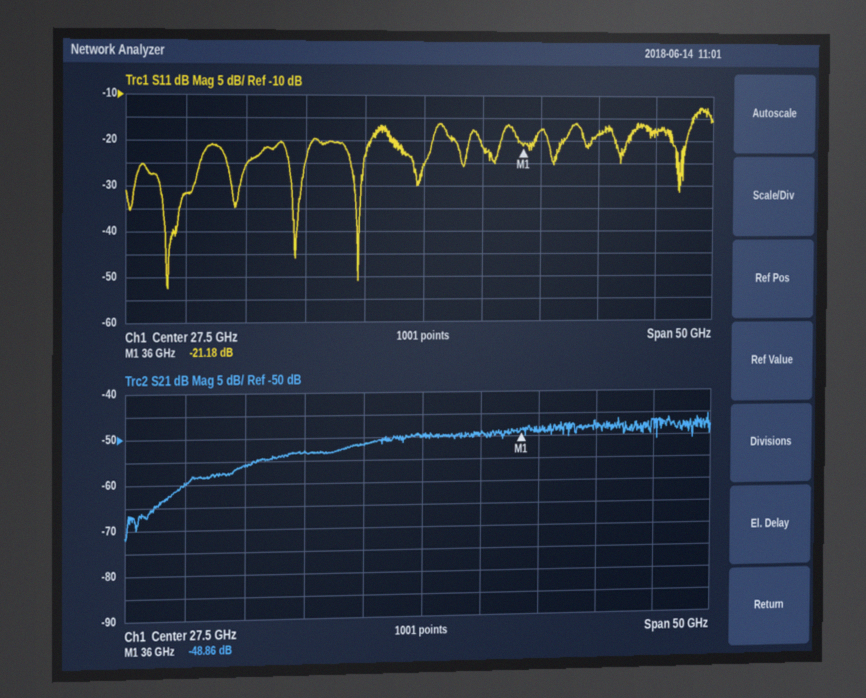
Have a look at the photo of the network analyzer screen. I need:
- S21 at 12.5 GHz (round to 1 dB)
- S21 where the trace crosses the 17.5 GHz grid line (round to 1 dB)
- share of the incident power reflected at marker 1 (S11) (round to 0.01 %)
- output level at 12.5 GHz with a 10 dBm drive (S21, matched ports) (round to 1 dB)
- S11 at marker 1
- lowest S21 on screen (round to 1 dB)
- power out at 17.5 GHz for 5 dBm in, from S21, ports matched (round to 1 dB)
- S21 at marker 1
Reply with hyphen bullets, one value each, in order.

- -56 dB
- -53 dB
- 0.76 %
- -46 dBm
- -21.18 dB
- -72 dB
- -48 dBm
- -48.86 dB
